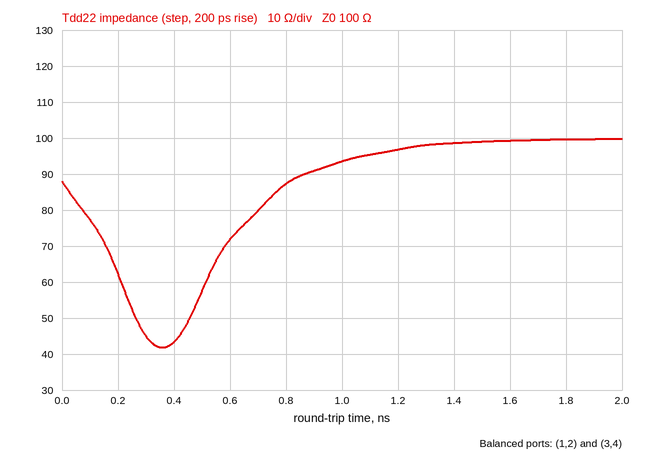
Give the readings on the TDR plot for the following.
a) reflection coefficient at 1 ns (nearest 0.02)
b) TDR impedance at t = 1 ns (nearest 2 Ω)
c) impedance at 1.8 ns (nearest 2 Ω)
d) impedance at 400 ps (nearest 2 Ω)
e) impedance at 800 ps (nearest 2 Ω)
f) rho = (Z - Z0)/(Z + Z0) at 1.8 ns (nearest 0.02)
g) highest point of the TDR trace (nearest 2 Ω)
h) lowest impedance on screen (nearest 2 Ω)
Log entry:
-0.04
94 Ω
100 Ω
44 Ω
88 Ω
0.00
100 Ω
42 Ω
